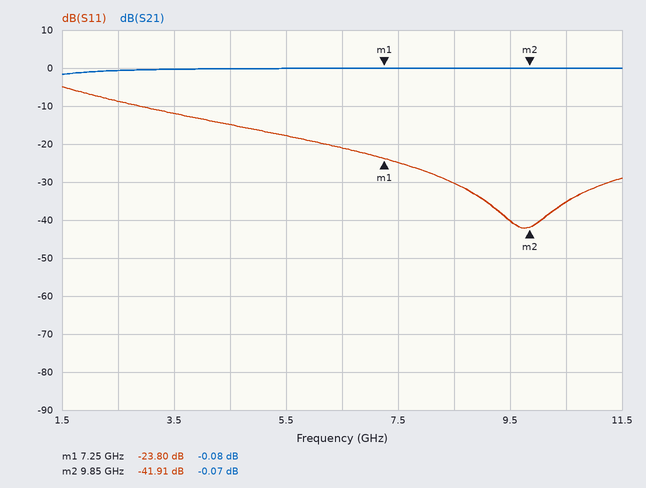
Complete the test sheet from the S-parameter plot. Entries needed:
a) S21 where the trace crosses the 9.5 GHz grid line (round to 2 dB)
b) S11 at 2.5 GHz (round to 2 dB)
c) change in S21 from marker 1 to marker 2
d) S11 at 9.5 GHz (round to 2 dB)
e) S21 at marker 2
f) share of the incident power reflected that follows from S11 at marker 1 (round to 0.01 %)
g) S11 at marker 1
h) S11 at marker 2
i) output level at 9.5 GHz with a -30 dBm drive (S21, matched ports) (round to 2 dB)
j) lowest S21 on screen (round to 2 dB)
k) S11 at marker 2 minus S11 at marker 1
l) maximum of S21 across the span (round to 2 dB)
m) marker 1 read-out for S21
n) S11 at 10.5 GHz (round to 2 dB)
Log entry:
0 dB
-8 dB
0.01 dB
-40 dB
-0.07 dB
0.42 %
-23.80 dB
-41.91 dB
-30 dBm
-2 dB
-18.11 dB
0 dB
-0.08 dB
-36 dB
